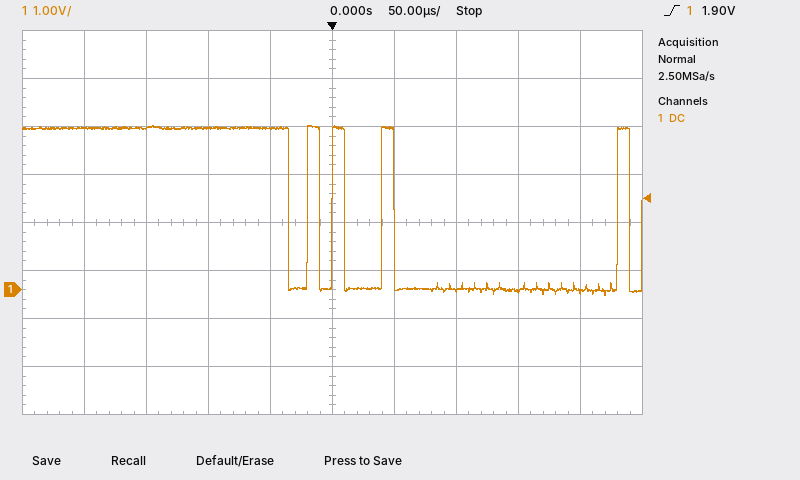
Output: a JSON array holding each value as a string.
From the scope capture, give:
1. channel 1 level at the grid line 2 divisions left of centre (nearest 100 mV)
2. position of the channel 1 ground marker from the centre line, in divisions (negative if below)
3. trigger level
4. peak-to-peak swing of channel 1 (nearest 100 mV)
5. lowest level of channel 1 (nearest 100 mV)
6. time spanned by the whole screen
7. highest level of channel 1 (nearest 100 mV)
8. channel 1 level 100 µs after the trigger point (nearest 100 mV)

["3.4 V", "-1.4 div", "1.90 V", "3.5 V", "-100 mV", "500 µs", "3.4 V", "0.0 V"]
